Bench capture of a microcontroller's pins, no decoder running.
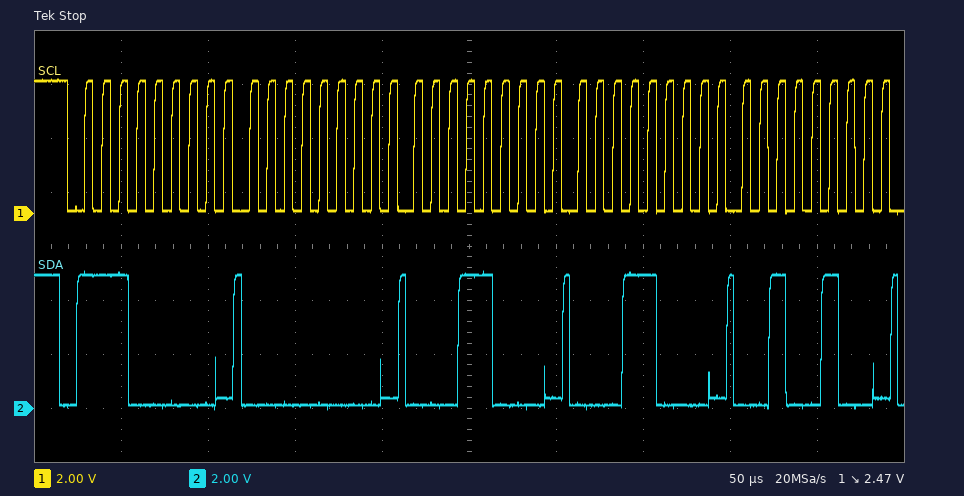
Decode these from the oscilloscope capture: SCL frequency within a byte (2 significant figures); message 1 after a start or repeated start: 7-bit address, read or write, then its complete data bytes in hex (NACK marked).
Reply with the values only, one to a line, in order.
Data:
100 kHz
0x70 write: 00 18 18 24
